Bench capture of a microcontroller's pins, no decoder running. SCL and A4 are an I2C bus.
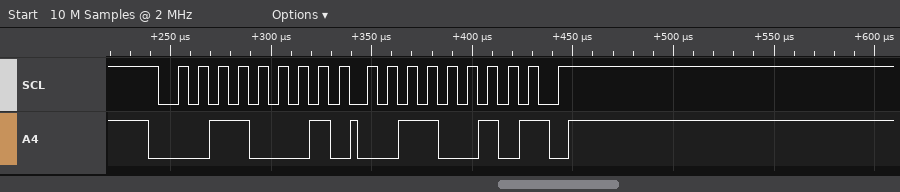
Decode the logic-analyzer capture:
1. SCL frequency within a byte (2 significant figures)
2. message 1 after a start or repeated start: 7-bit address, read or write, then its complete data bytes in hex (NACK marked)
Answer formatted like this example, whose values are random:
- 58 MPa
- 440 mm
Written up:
- 100 kHz
- 0x18 read: 32 NACK
